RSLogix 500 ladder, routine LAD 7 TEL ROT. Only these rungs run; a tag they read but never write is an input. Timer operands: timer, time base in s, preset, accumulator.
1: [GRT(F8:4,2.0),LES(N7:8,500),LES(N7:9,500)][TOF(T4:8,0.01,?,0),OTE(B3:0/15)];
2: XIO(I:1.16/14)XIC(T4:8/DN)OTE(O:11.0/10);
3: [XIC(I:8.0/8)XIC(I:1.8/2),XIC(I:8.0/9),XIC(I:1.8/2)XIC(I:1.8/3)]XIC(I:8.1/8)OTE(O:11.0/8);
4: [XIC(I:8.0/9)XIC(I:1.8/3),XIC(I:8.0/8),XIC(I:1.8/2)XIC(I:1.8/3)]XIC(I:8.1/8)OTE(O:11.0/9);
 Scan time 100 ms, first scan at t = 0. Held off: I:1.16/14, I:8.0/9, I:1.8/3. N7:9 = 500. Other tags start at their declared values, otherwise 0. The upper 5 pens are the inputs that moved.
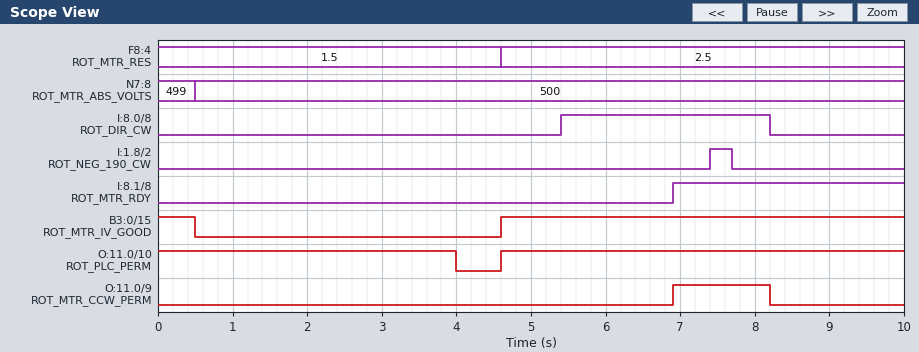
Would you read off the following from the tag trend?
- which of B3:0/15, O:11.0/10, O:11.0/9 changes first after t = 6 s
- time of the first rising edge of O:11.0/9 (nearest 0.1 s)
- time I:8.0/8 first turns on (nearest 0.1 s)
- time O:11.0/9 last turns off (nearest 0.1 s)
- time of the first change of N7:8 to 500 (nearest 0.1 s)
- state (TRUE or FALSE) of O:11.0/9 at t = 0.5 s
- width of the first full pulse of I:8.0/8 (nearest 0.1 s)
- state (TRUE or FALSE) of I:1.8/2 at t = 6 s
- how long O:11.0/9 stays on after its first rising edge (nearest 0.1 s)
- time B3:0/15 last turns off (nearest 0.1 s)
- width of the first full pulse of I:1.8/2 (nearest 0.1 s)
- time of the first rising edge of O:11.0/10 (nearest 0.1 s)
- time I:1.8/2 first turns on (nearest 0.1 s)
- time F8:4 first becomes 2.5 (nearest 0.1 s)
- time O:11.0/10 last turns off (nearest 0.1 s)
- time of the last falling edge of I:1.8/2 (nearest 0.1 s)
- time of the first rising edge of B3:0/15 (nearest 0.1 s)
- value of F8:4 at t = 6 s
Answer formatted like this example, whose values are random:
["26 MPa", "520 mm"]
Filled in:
["O:11.0/9", "6.9 s", "5.4 s", "8.2 s", "0.5 s", "FALSE", "2.8 s", "FALSE", "1.3 s", "0.5 s", "0.3 s", "4.6 s", "7.4 s", "4.6 s", "4.0 s", "7.7 s", "4.6 s", "2.5"]
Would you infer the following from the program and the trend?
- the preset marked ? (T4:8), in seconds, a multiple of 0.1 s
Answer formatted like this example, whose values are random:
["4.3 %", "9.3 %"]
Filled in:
["3.5 s"]
